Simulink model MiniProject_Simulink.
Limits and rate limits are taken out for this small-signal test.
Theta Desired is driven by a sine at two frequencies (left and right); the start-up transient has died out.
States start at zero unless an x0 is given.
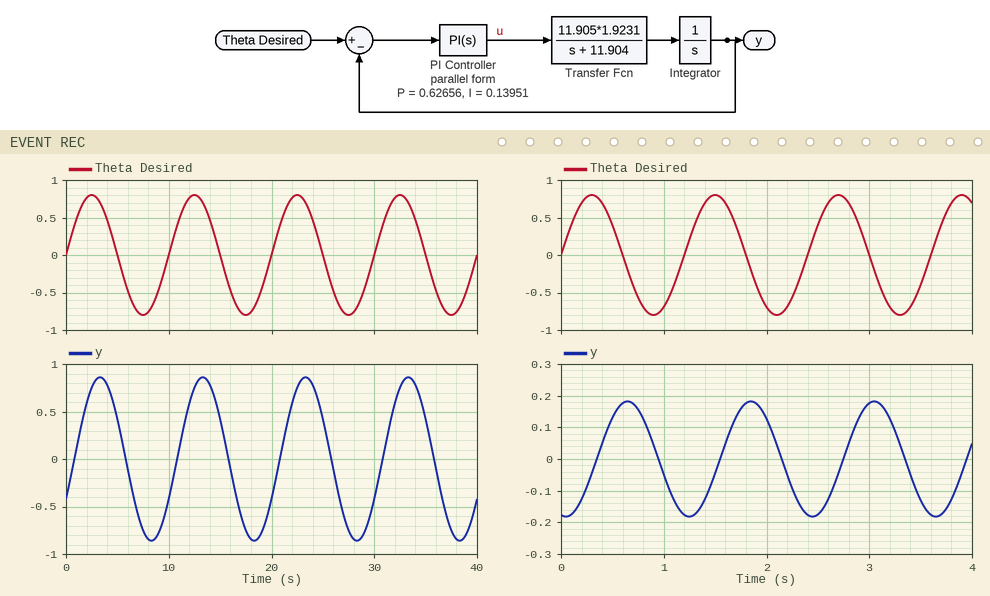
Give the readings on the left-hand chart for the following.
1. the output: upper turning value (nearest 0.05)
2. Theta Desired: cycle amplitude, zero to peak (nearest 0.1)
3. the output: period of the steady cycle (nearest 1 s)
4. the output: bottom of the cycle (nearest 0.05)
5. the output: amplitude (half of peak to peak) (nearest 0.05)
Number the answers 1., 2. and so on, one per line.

1. 0.85
2. 0.8
3. 10 s
4. -0.85
5. 0.85
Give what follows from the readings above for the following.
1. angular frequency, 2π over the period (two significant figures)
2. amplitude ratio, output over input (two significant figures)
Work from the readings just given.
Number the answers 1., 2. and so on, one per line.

1. 0.63 rad/s
2. 1.1
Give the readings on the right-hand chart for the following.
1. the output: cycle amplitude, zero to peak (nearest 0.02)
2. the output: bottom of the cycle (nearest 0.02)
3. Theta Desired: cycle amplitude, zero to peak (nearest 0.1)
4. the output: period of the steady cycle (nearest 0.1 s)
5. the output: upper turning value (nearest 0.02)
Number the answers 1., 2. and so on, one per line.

1. 0.18
2. -0.18
3. 0.8
4. 1.2 s
5. 0.18
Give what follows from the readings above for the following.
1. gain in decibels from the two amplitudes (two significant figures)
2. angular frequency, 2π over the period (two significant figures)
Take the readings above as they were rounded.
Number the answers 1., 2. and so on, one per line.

1. -13 dB
2. 5.2 rad/s
